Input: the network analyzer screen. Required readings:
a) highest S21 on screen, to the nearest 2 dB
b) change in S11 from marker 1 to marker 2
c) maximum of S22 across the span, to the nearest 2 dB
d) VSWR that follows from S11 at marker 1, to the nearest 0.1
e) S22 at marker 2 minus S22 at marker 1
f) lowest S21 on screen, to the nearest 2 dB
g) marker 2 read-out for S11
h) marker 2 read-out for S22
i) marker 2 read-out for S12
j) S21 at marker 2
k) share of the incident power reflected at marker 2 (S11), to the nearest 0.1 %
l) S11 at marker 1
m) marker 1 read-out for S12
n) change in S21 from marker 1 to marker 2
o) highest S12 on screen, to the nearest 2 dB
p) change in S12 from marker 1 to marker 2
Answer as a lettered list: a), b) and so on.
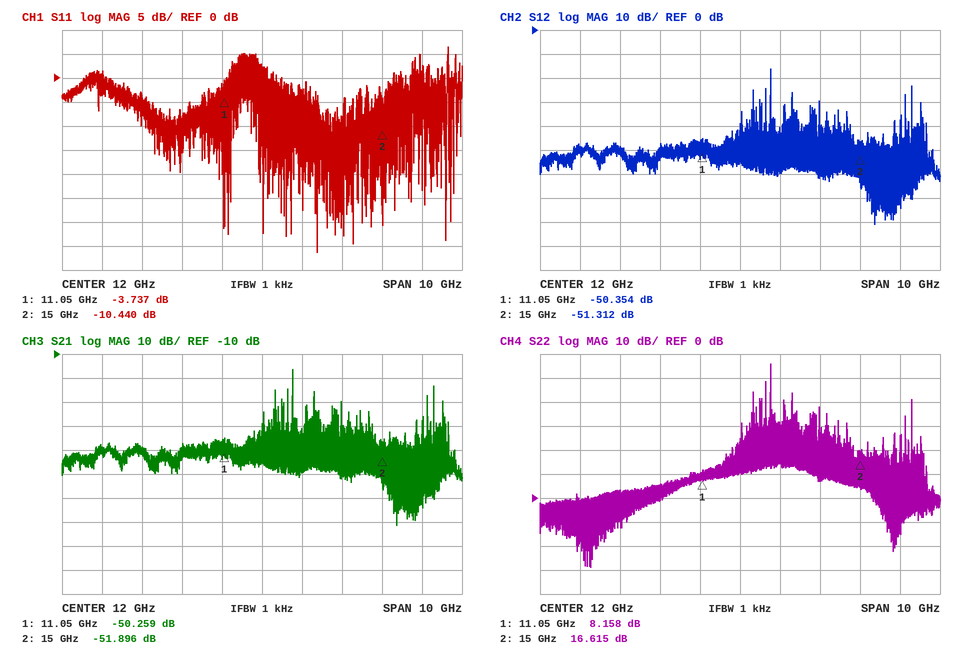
a) -16 dB
b) -6.703 dB
c) 56 dB
d) 4.7
e) 8.457 dB
f) -82 dB
g) -10.440 dB
h) 16.615 dB
i) -51.312 dB
j) -51.896 dB
k) 9.0 %
l) -3.737 dB
m) -50.354 dB
n) -1.637 dB
o) -16 dB
p) -0.958 dB
